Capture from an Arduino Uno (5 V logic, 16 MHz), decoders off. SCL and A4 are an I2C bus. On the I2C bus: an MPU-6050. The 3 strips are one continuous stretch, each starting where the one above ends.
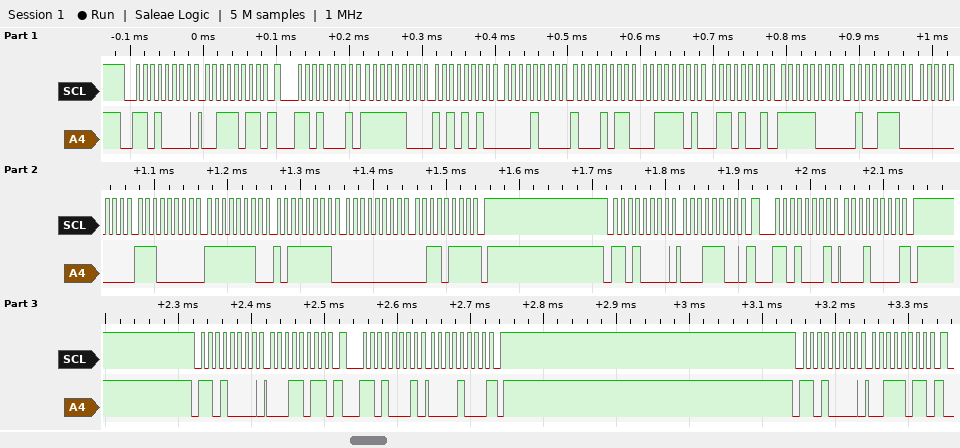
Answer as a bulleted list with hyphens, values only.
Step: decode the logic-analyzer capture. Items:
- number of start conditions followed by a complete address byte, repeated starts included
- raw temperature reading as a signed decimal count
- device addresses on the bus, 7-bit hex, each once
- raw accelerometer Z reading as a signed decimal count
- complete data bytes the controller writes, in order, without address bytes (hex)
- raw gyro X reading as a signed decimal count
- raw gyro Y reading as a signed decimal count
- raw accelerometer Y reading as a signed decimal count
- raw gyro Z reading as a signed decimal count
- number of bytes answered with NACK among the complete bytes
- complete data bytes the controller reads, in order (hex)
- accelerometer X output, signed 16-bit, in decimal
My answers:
- 7
- -1970
- 0x68
- 15721
- 3B 1C 1B 3B
- 224
- -321
- 2187
- 55
- 3
- FC AA 08 8B 3D 69 F8 4E 00 E0 FE BF 00 37 10 08
- -854
